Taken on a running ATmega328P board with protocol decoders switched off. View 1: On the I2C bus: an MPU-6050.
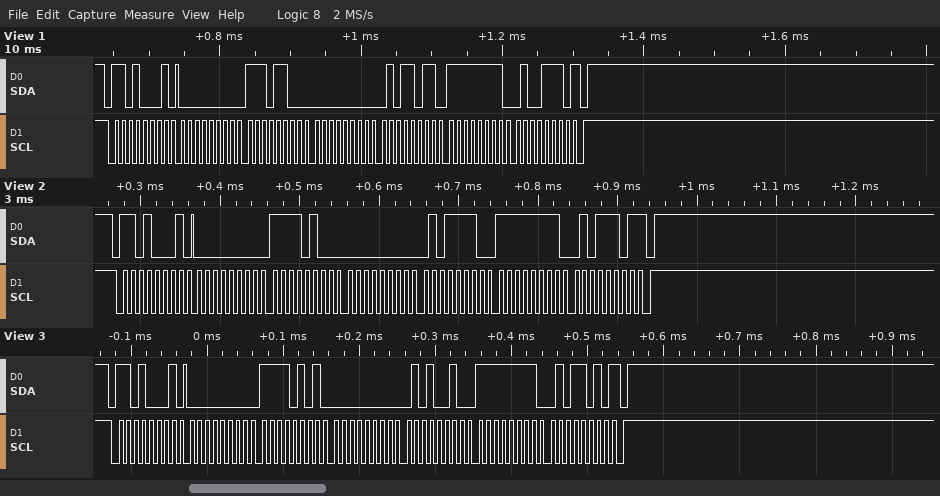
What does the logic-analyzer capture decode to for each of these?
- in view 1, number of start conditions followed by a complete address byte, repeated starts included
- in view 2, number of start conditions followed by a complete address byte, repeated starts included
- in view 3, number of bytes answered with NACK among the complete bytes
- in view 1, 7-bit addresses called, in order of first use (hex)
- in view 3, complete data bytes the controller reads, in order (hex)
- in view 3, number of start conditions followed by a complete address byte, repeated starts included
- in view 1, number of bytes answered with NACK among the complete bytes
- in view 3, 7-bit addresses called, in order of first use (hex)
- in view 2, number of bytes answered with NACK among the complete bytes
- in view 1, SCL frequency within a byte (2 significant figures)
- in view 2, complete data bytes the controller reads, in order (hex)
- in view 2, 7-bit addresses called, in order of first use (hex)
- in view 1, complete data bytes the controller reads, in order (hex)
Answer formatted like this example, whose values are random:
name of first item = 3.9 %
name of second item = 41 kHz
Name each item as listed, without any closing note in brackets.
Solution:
in view 1, number of start conditions followed by a complete address byte, repeated starts included = 1
in view 2, number of start conditions followed by a complete address byte, repeated starts included = 1
in view 3, number of bytes answered with NACK among the complete bytes = 1
in view 1, 7-bit addresses called, in order of first use = 0x68
in view 3, complete data bytes the controller reads, in order = 00 F5 00 52 FF 5A
in view 3, number of start conditions followed by a complete address byte, repeated starts included = 1
in view 1, number of bytes answered with NACK among the complete bytes = 1
in view 3, 7-bit addresses called, in order of first use = 0x68
in view 2, number of bytes answered with NACK among the complete bytes = 1
in view 1, SCL frequency within a byte = 100 kHz
in view 2, complete data bytes the controller reads, in order = 00 F4 00 5E FF 5D
in view 2, 7-bit addresses called, in order of first use = 0x68
in view 1, complete data bytes the controller reads, in order = 00 EC 00 5B FF 4E
